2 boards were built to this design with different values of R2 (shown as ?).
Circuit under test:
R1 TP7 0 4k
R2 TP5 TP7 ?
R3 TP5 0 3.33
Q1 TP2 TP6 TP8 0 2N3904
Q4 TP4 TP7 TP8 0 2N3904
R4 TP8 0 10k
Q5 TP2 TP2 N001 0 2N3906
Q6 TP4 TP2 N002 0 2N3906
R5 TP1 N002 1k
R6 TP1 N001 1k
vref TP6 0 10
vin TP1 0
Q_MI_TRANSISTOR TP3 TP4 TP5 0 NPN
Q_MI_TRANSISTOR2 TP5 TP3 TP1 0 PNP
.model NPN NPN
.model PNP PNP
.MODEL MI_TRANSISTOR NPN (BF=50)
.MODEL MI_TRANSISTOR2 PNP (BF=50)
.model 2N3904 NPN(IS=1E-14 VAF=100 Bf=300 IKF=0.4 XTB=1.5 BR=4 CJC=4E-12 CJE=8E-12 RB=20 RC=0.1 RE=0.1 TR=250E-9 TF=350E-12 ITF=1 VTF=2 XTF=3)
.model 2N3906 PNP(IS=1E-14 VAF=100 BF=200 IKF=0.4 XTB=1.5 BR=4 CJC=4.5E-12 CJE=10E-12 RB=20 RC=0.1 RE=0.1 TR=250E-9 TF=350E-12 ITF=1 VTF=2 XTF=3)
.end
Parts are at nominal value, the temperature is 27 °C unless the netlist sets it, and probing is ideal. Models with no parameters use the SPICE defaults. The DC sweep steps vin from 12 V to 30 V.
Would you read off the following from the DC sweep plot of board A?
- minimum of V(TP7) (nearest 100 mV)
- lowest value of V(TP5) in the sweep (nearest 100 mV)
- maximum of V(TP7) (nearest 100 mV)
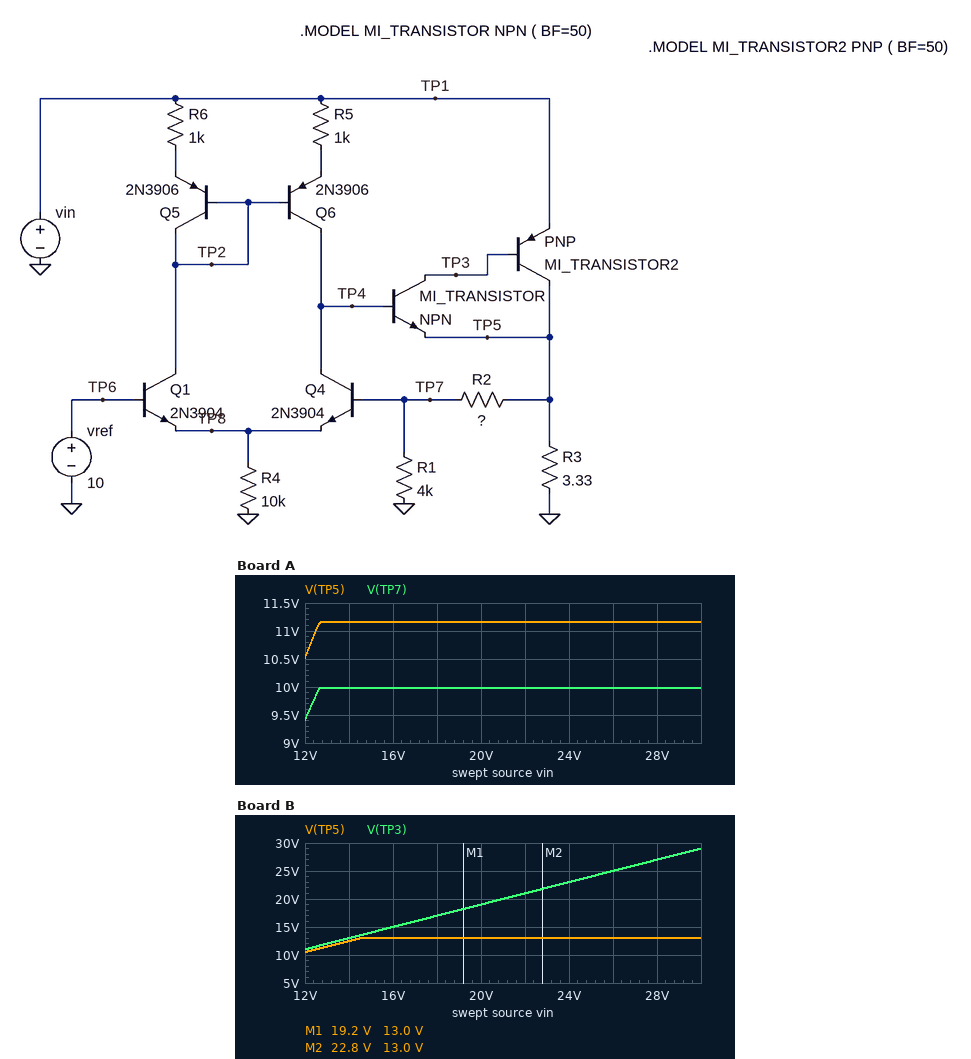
9.4 V
10.5 V
10.0 V
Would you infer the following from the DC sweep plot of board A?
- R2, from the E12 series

470 Ω
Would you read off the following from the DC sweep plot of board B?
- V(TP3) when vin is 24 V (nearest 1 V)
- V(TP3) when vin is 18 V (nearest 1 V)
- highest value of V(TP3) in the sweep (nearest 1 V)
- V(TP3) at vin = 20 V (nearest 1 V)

23 V
17 V
29 V
19 V
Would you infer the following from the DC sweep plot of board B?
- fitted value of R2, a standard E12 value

1.2 kΩ
